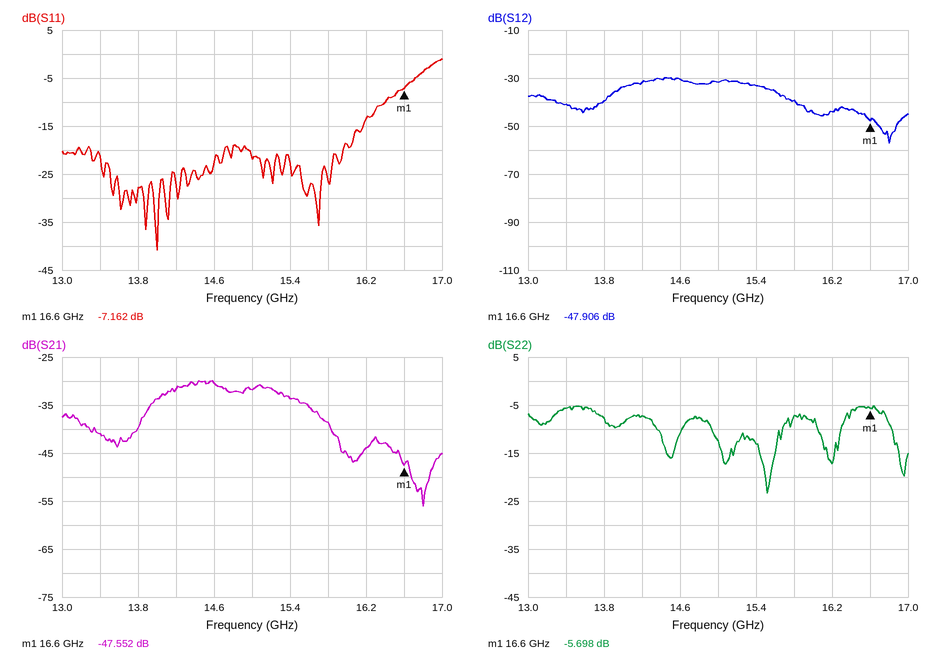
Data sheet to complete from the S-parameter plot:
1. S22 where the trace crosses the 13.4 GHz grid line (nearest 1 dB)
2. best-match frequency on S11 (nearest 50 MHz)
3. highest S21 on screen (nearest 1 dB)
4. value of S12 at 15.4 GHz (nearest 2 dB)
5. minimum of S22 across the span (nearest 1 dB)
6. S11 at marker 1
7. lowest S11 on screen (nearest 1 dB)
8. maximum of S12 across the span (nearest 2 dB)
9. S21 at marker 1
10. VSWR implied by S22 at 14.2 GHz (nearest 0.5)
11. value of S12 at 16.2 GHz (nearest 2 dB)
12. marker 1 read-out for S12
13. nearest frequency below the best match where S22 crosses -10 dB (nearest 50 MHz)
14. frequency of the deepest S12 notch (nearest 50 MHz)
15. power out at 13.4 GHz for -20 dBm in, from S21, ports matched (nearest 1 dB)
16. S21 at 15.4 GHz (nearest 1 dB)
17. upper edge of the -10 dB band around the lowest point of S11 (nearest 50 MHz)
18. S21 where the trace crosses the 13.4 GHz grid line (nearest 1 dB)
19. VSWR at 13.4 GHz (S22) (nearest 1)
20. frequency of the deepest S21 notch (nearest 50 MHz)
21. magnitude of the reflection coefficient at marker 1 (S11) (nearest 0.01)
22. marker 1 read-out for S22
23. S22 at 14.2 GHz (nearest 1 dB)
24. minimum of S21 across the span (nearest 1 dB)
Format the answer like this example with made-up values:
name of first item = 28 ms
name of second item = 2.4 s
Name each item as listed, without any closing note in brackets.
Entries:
S22 where the trace crosses the 13.4 GHz grid line = -6 dB
best-match frequency on S11 = 14.00 GHz
highest S21 on screen = -30 dB
value of S12 at 15.4 GHz = -34 dB
minimum of S22 across the span = -23 dB
S11 at marker 1 = -7.162 dB
lowest S11 on screen = -41 dB
maximum of S12 across the span = -30 dB
S21 at marker 1 = -47.552 dB
VSWR implied by S22 at 14.2 GHz = 2.5
value of S12 at 16.2 GHz = -44 dB
marker 1 read-out for S12 = -47.906 dB
nearest frequency below the best match where S22 crosses -10 dB = 14.95 GHz
frequency of the deepest S12 notch = 16.80 GHz
power out at 13.4 GHz for -20 dBm in, from S21, ports matched = -61 dBm
S21 at 15.4 GHz = -34 dB
upper edge of the -10 dB band around the lowest point of S11 = 16.40 GHz
S21 where the trace crosses the 13.4 GHz grid line = -41 dB
VSWR at 13.4 GHz (S22) = 3
frequency of the deepest S21 notch = 16.80 GHz
magnitude of the reflection coefficient at marker 1 (S11) = 0.44
marker 1 read-out for S22 = -5.698 dB
S22 at 14.2 GHz = -7 dB
minimum of S21 across the span = -56 dB
